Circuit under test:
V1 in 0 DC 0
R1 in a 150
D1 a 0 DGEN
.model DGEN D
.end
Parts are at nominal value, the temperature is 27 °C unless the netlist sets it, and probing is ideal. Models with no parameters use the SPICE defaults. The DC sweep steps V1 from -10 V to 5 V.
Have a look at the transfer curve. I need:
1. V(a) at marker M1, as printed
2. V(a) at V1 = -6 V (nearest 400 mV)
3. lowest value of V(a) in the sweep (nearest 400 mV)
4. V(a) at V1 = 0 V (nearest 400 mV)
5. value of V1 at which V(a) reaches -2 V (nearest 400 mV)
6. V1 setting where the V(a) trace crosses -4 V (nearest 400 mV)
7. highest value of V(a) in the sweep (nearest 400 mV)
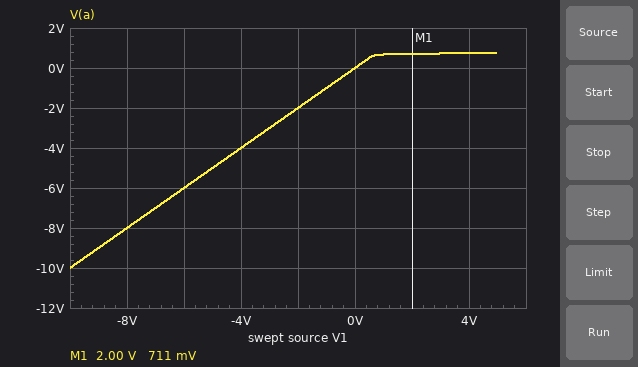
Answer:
711 mV
-6.0 V
-10.0 V
0 V
-2.0 V
-4.0 V
800 mV
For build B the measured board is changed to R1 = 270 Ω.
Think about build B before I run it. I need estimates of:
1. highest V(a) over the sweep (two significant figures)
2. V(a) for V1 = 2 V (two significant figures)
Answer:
730 mV
700 mV
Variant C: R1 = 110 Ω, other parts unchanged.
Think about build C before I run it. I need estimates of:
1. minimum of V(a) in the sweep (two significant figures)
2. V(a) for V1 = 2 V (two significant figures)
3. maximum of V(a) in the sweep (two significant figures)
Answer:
-10 V
720 mV
750 mV
